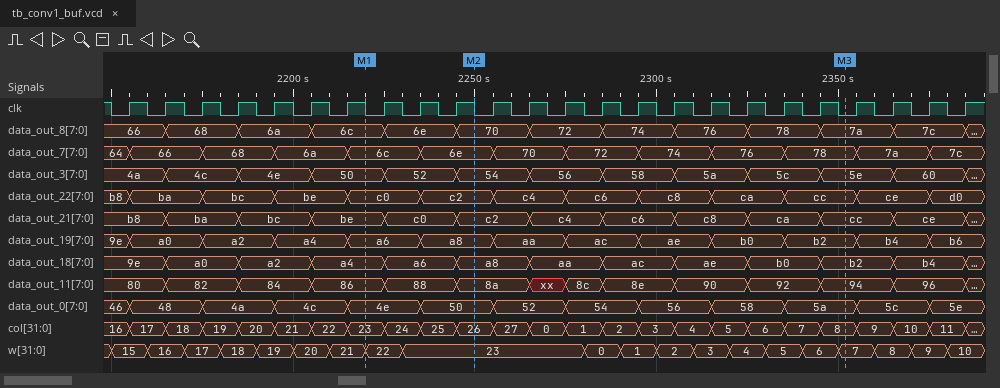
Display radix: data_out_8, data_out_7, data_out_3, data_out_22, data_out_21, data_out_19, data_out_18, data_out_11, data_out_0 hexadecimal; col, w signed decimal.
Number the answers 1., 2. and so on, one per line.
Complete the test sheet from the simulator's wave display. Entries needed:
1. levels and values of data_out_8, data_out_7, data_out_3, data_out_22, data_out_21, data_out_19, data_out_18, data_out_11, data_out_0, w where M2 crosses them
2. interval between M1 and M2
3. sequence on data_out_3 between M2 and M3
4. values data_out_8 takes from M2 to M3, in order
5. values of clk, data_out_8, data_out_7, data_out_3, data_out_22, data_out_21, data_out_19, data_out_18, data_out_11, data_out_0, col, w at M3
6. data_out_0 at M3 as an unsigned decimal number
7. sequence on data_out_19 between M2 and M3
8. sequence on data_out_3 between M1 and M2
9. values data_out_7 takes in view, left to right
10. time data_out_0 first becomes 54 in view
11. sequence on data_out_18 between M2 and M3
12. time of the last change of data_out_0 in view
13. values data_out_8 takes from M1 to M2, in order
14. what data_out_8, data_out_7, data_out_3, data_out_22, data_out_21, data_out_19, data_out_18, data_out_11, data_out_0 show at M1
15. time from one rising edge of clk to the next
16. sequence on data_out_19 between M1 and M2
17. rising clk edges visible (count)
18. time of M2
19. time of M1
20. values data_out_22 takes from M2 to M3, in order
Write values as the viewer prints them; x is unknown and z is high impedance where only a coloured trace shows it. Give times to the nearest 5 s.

1. data_out_8=70, data_out_7=6e, data_out_3=54, data_out_22=c2, data_out_21=c2, data_out_19=a8, data_out_18=a8, data_out_11=8a, data_out_0=50, w=23
2. 30 s
3. 54, 56, 58, 5a, 5c, 5e
4. 70, 72, 74, 76, 78, 7a
5. clk=0, data_out_8=7a, data_out_7=78, data_out_3=5e, data_out_22=cc, data_out_21=cc, data_out_19=b2, data_out_18=b2, data_out_11=94, data_out_0=5a, col=8, w=7
6. 90
7. a8, aa, ac, ae, b0, b2
8. 50, 52, 54
9. 64, 66, 68, 6a, 6c, 6e, 70, 72, 74, 76, 78, 7a, 7c
10. 2275 s
11. a8, aa, ac, ae, b0, b2
12. 2375 s
13. 6c, 6e, 70
14. data_out_8=6c, data_out_7=6c, data_out_3=50, data_out_22=c0, data_out_21=be, data_out_19=a6, data_out_18=a4, data_out_11=86, data_out_0=4e
15. 10 s
16. a6, a8
17. 24
18. 2250 s
19. 2220 s
20. c2, c4, c6, c8, ca, cc
